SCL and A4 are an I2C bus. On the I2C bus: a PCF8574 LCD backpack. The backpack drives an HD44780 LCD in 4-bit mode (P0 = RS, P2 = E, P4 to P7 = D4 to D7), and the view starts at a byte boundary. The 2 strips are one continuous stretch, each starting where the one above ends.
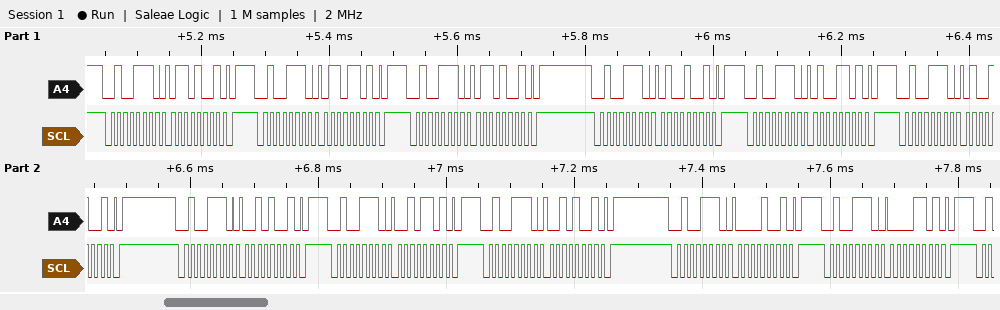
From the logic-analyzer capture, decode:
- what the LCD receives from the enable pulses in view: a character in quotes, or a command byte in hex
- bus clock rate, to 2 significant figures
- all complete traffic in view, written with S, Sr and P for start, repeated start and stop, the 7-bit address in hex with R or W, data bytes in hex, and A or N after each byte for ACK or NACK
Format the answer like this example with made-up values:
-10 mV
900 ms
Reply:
'd'
100 kHz
S 27W A 69 A P S 27W A 6D A P S 27W A 69 A P S 27W A 49 A P S 27W A 4D A P S 27W A 49 A P S 27W A 29 A P S 27W A 2D A P S 27W A 29 A P S 27W A 09 A P S 27W A 0D A P
